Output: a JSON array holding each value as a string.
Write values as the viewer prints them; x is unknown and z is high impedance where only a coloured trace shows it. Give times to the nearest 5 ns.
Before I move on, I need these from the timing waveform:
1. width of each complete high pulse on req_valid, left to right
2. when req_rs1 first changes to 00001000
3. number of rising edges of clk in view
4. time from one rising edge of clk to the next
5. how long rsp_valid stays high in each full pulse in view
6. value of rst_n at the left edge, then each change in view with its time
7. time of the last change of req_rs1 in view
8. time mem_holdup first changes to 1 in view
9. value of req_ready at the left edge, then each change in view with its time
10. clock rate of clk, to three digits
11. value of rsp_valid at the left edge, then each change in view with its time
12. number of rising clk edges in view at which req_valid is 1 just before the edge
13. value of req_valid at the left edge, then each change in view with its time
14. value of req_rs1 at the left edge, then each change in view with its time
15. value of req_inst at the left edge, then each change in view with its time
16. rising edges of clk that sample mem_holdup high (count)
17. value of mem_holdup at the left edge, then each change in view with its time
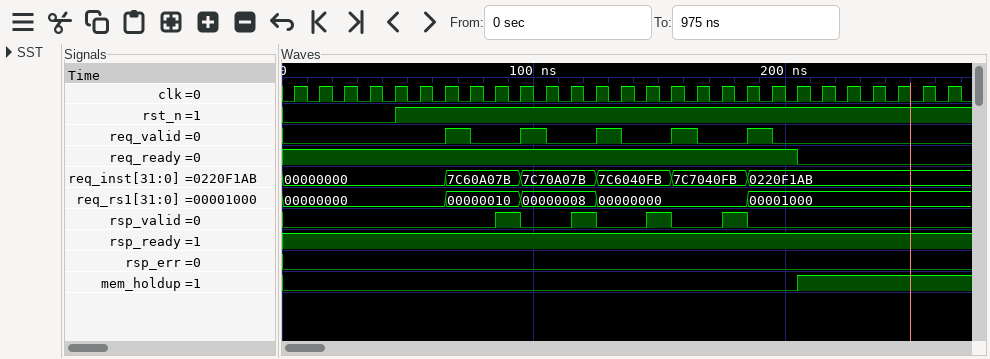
["10 ns, 10 ns, 10 ns, 10 ns, 10 ns", "185 ns", "27", "10 ns", "10 ns, 10 ns, 10 ns, 10 ns", "0, 1 at 45 ns", "185 ns", "205 ns", "1, 0 at 205 ns", "100 MHz", "0, 1 at 85 ns, 0 at 95 ns, 1 at 115 ns, 0 at 125 ns, 1 at 145 ns, 0 at 155 ns, 1 at 175 ns, 0 at 185 ns", "5", "0, 1 at 65 ns, 0 at 75 ns, 1 at 95 ns, 0 at 105 ns, 1 at 125 ns, 0 at 135 ns, 1 at 155 ns, 0 at 165 ns, 1 at 185 ns, 0 at 195 ns", "00000000, 00000010 at 65 ns, 00000008 at 95 ns, 00000000 at 125 ns, 00001000 at 185 ns", "00000000, 7C60A07B at 65 ns, 7C70A07B at 95 ns, 7C6040FB at 125 ns, 7C7040FB at 155 ns, 0220F1AB at 185 ns", "6", "0, 1 at 205 ns"]
